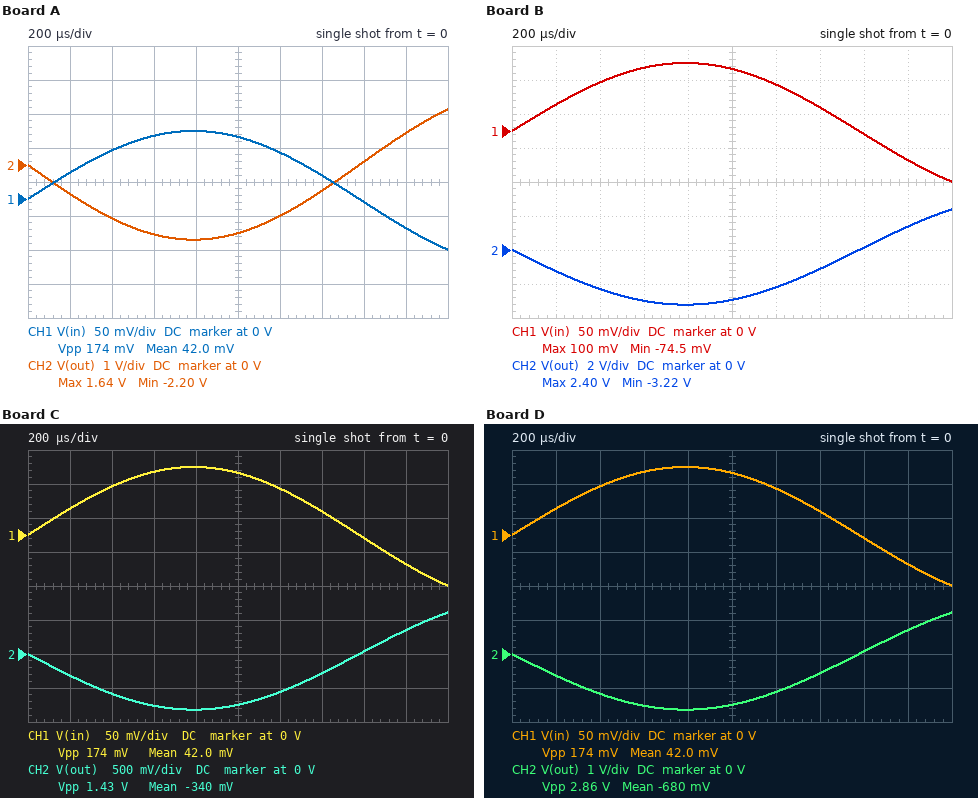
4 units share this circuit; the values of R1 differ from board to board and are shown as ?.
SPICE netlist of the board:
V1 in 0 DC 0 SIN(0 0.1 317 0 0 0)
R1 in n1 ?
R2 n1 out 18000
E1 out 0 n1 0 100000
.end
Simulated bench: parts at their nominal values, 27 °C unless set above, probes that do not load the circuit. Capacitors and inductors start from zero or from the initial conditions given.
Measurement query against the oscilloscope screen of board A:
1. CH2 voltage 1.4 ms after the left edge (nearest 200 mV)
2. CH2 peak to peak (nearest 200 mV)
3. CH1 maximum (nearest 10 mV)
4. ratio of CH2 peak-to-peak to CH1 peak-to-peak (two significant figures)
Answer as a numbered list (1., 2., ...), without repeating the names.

1. -800 mV
2. 3.8 V
3. 100 mV
4. 22
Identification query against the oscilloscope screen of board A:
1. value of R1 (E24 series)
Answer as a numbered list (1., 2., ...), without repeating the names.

1. 820 Ω
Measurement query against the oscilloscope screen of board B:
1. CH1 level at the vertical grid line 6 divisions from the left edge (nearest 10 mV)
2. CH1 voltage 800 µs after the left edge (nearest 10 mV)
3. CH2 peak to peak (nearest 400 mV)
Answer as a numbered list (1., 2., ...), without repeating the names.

1. 70 mV
2. 100 mV
3. 5.6 V
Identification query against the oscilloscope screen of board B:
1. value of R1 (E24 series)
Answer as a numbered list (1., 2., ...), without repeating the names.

1. 560 Ω
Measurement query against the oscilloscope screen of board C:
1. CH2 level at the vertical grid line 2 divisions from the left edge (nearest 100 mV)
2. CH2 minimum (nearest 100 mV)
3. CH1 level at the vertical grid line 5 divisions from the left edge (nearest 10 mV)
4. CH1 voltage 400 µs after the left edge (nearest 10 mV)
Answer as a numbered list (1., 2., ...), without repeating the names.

1. -600 mV
2. -800 mV
3. 90 mV
4. 70 mV
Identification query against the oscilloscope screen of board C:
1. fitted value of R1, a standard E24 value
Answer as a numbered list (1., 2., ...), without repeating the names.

1. 2.2 kΩ
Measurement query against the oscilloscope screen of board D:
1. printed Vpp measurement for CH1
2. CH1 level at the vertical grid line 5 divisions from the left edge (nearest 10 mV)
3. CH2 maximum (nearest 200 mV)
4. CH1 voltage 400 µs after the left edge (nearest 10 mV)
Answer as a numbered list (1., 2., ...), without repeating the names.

1. 174 mV
2. 90 mV
3. 1.2 V
4. 70 mV
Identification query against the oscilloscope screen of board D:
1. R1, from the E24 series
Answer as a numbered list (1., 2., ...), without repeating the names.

1. 1.1 kΩ
